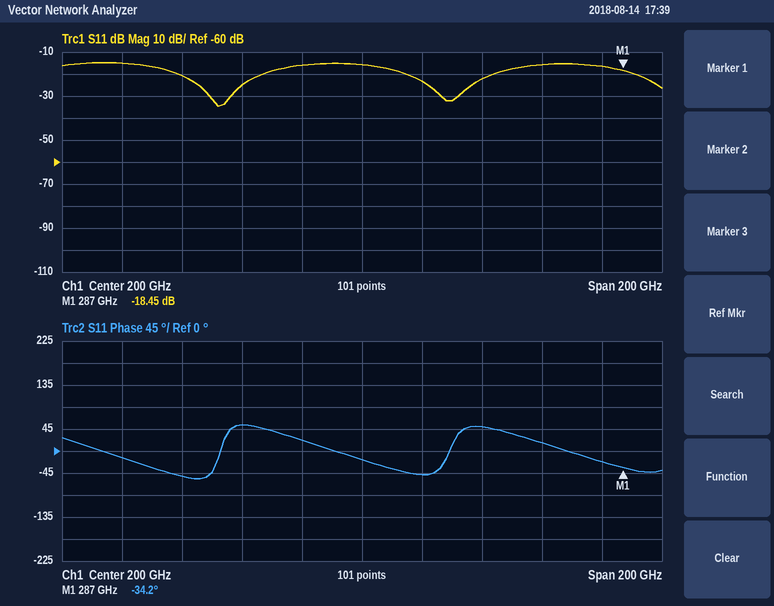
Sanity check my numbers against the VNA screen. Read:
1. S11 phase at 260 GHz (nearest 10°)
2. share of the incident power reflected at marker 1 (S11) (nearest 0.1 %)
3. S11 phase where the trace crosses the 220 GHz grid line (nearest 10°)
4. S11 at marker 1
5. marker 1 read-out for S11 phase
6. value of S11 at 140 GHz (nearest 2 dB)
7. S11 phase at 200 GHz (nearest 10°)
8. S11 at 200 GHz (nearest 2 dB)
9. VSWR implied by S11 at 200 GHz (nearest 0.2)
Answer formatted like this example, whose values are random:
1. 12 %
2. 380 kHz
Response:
1. 20°
2. 1.4 %
3. -50°
4. -18.45 dB
5. -34.2°
6. -20 dB
7. -20°
8. -16 dB
9. 1.4
